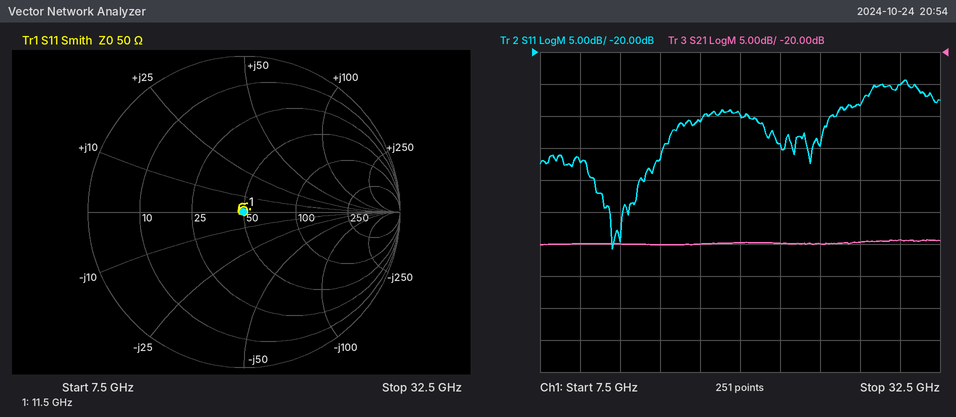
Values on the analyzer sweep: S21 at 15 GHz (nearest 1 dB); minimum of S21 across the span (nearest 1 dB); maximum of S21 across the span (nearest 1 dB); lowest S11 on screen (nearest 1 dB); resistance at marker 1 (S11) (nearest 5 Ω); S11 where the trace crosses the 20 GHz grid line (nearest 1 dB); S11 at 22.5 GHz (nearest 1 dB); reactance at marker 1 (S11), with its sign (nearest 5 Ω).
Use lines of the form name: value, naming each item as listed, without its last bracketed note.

S21 at 15 GHz: -50 dB
minimum of S21 across the span: -50 dB
maximum of S21 across the span: -49 dB
lowest S11 on screen: -51 dB
resistance at marker 1 (S11): 50 Ω
S11 where the trace crosses the 20 GHz grid line: -30 dB
S11 at 22.5 GHz: -34 dB
reactance at marker 1 (S11), with its sign: 0 Ω
